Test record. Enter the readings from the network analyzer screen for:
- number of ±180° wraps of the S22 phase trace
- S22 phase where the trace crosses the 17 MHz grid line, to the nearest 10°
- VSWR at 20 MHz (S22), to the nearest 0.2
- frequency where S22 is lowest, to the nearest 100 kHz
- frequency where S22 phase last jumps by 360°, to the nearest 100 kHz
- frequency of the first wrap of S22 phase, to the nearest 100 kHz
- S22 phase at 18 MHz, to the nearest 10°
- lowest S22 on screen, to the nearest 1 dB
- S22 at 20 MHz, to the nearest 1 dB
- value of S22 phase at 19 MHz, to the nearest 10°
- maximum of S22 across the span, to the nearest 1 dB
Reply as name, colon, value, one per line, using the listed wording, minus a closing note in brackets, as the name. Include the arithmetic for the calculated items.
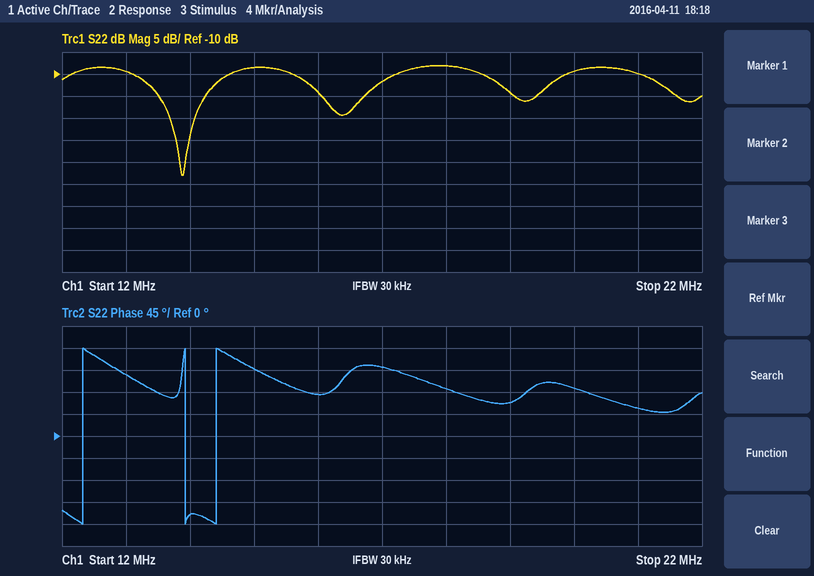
number of ±180° wraps of the S22 phase trace: 3
S22 phase where the trace crosses the 17 MHz grid line, to the nearest 10°: 140°
VSWR at 20 MHz (S22), to the nearest 0.2: |Γ| = 10^(-9/20) = 0.3548; VSWR = (1 + 0.3548)/(1 − 0.3548) ≈ 2.10, so 2.0 to the nearest 0.2
frequency where S22 is lowest, to the nearest 100 kHz: 13.9 MHz
frequency where S22 phase last jumps by 360°, to the nearest 100 kHz: 14.4 MHz
frequency of the first wrap of S22 phase, to the nearest 100 kHz: 12.3 MHz
S22 phase at 18 MHz, to the nearest 10°: 100°
lowest S22 on screen, to the nearest 1 dB: -33 dB
S22 at 20 MHz, to the nearest 1 dB: -9 dB
value of S22 phase at 19 MHz, to the nearest 10°: 70°
maximum of S22 across the span, to the nearest 1 dB: -8 dB
